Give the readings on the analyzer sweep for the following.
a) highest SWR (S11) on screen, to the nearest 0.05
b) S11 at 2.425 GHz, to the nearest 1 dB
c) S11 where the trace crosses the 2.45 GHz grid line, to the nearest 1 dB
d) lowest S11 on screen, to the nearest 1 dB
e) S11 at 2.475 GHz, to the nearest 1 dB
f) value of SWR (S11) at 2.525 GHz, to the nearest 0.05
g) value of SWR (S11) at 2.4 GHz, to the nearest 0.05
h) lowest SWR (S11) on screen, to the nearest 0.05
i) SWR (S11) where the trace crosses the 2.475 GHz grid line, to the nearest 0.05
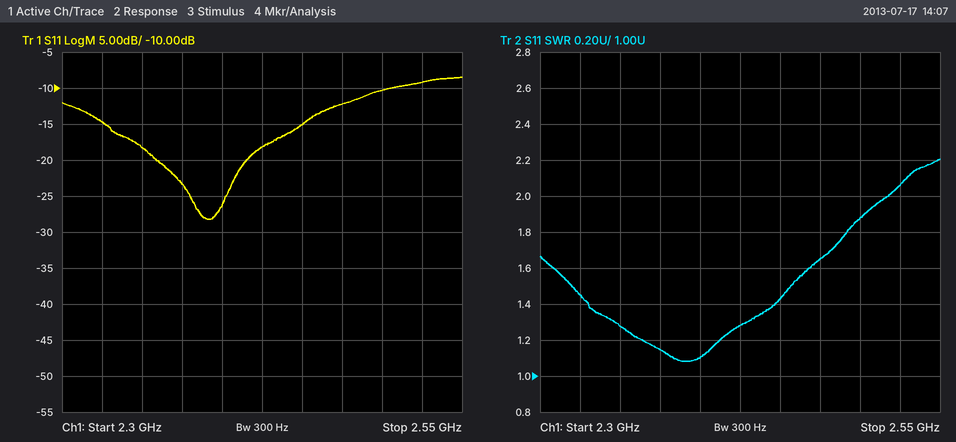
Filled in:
2.20
-18 dB
-15 dB
-28 dB
-12 dB
2.05
1.10
1.10
1.65
